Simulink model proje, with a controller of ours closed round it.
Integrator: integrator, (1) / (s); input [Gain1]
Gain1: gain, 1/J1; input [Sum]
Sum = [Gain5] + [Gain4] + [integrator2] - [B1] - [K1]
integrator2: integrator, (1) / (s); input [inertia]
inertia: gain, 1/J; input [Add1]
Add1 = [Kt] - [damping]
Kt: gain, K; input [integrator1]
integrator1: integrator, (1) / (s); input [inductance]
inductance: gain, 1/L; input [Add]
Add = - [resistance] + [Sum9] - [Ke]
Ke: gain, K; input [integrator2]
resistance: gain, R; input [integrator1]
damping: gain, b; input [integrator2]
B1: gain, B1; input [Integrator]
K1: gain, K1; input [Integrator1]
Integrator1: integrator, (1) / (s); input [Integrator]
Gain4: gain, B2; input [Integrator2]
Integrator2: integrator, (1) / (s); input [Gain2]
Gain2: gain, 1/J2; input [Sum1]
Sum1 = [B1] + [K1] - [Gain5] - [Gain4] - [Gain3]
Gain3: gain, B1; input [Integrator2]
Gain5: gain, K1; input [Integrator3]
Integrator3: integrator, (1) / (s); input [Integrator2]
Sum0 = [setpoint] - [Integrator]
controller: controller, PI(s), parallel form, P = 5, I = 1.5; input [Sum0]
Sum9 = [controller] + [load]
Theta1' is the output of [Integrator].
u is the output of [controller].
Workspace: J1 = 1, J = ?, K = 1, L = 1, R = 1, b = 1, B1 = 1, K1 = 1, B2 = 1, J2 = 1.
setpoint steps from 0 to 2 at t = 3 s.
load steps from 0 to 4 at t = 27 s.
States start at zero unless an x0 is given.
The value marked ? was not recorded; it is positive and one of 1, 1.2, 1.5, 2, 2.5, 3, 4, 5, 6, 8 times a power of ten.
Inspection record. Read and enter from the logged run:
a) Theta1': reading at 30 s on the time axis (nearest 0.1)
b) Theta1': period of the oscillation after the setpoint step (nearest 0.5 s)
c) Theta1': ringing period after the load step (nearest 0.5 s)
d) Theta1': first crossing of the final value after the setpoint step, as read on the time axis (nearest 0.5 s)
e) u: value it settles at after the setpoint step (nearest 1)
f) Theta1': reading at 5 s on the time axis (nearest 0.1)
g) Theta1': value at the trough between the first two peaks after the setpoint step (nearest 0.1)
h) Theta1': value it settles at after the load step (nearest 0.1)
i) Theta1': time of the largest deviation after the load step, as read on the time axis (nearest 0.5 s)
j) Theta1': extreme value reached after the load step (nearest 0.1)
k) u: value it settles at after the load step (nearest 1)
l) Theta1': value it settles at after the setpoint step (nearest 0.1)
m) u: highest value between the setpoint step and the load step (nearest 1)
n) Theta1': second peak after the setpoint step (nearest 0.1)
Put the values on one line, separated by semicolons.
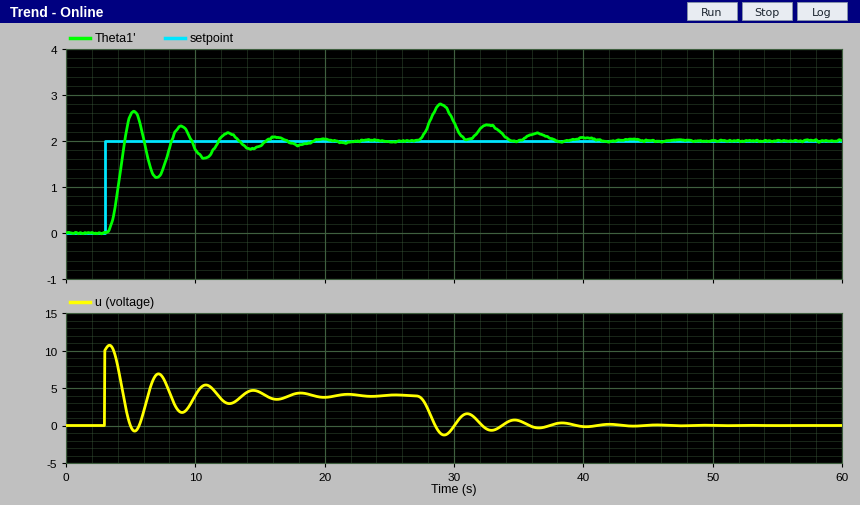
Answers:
2.4; 3.5 s; 3.5 s; 4.5 s; 4; 2.6; 1.2; 2.0; 29.0 s; 2.8; 0; 2.0; 11; 2.3
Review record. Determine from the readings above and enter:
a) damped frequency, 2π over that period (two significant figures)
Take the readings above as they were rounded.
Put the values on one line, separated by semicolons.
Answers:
1.8 rad/s
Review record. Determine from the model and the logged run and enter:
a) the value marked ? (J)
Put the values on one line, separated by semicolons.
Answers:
0.8
